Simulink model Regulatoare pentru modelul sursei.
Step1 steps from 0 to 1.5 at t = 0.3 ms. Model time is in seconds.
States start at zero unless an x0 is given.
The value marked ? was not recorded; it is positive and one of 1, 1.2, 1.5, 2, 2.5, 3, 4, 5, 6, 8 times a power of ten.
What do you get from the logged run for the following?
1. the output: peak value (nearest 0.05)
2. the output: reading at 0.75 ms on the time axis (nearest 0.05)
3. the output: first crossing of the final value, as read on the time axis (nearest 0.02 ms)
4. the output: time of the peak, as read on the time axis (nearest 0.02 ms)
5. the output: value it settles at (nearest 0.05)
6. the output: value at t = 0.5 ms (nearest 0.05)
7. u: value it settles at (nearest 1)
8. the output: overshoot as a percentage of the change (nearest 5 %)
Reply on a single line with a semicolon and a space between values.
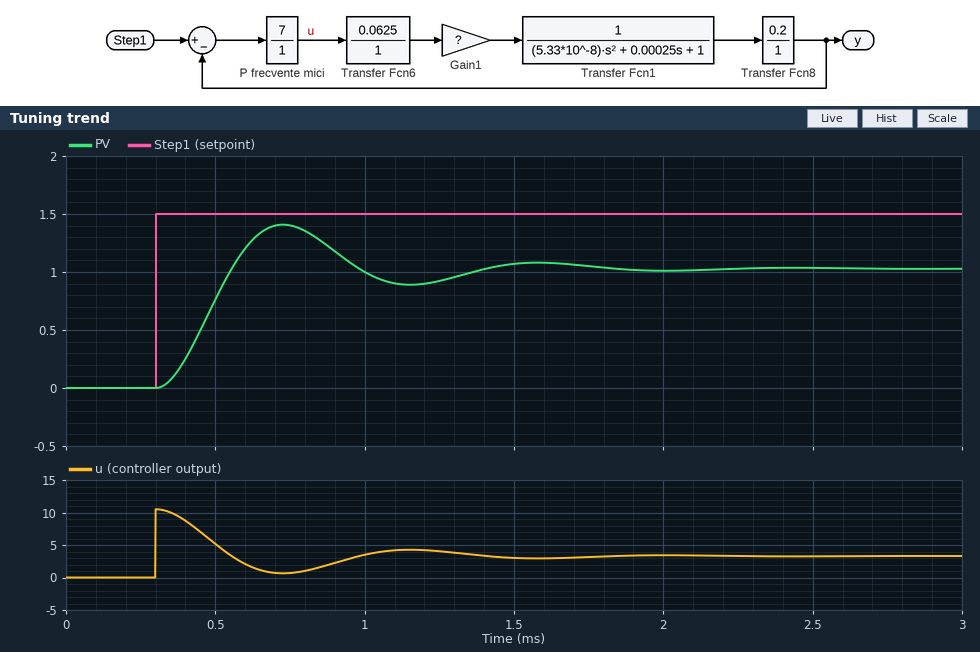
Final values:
1.40; 1.40; 0.56 ms; 0.72 ms; 1.05; 0.75; 3; 35 %
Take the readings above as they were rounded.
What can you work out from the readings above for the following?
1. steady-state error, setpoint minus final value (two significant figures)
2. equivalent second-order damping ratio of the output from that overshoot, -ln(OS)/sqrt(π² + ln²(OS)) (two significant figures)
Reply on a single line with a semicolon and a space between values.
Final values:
0.45; 0.32
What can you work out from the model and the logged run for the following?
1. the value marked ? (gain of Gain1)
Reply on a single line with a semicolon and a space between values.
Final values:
25
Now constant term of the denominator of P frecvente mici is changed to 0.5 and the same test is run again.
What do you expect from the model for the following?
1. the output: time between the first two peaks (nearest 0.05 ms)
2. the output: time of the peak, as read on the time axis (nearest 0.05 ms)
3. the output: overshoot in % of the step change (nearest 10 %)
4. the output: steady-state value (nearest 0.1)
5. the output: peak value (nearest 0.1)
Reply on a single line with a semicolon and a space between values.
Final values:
0.65 ms; 0.60 ms; 50 %; 1.2; 1.8
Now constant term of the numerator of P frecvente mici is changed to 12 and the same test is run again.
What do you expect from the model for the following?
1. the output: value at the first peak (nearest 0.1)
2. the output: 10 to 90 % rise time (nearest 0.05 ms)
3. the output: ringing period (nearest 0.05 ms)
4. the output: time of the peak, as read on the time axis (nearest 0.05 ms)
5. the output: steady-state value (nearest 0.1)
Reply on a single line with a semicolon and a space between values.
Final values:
1.7; 0.15 ms; 0.70 ms; 0.65 ms; 1.2
